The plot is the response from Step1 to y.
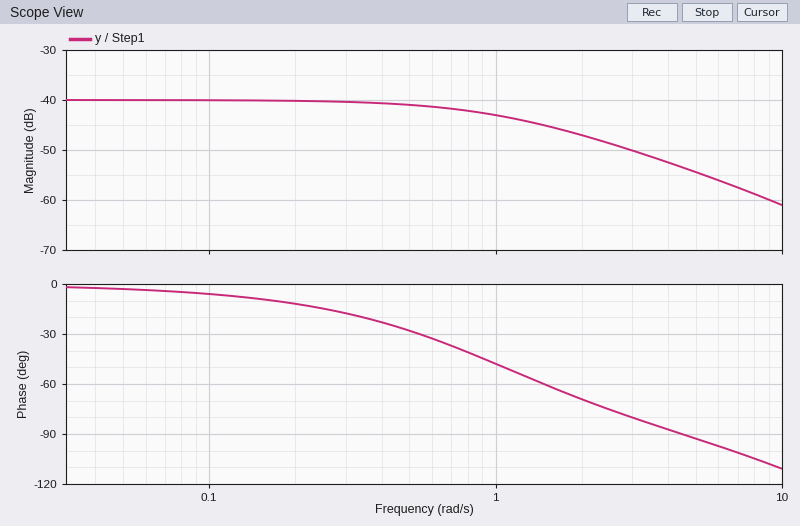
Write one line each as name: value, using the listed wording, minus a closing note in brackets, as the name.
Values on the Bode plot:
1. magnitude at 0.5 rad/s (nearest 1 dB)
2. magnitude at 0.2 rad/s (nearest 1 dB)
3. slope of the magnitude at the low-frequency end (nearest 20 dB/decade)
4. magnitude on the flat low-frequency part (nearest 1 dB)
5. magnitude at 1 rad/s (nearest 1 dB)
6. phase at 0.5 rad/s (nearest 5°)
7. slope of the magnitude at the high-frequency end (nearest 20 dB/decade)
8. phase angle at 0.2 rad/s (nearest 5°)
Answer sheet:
magnitude at 0.5 rad/s: -41 dB
magnitude at 0.2 rad/s: -40 dB
slope of the magnitude at the low-frequency end: 0 dB/decade
magnitude on the flat low-frequency part: -40 dB
magnitude at 1 rad/s: -43 dB
phase at 0.5 rad/s: -30°
slope of the magnitude at the high-frequency end: -20 dB/decade
phase angle at 0.2 rad/s: -10°
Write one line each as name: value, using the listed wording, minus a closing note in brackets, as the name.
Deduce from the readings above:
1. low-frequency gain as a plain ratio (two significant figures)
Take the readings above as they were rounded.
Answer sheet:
low-frequency gain as a plain ratio: 0.010
